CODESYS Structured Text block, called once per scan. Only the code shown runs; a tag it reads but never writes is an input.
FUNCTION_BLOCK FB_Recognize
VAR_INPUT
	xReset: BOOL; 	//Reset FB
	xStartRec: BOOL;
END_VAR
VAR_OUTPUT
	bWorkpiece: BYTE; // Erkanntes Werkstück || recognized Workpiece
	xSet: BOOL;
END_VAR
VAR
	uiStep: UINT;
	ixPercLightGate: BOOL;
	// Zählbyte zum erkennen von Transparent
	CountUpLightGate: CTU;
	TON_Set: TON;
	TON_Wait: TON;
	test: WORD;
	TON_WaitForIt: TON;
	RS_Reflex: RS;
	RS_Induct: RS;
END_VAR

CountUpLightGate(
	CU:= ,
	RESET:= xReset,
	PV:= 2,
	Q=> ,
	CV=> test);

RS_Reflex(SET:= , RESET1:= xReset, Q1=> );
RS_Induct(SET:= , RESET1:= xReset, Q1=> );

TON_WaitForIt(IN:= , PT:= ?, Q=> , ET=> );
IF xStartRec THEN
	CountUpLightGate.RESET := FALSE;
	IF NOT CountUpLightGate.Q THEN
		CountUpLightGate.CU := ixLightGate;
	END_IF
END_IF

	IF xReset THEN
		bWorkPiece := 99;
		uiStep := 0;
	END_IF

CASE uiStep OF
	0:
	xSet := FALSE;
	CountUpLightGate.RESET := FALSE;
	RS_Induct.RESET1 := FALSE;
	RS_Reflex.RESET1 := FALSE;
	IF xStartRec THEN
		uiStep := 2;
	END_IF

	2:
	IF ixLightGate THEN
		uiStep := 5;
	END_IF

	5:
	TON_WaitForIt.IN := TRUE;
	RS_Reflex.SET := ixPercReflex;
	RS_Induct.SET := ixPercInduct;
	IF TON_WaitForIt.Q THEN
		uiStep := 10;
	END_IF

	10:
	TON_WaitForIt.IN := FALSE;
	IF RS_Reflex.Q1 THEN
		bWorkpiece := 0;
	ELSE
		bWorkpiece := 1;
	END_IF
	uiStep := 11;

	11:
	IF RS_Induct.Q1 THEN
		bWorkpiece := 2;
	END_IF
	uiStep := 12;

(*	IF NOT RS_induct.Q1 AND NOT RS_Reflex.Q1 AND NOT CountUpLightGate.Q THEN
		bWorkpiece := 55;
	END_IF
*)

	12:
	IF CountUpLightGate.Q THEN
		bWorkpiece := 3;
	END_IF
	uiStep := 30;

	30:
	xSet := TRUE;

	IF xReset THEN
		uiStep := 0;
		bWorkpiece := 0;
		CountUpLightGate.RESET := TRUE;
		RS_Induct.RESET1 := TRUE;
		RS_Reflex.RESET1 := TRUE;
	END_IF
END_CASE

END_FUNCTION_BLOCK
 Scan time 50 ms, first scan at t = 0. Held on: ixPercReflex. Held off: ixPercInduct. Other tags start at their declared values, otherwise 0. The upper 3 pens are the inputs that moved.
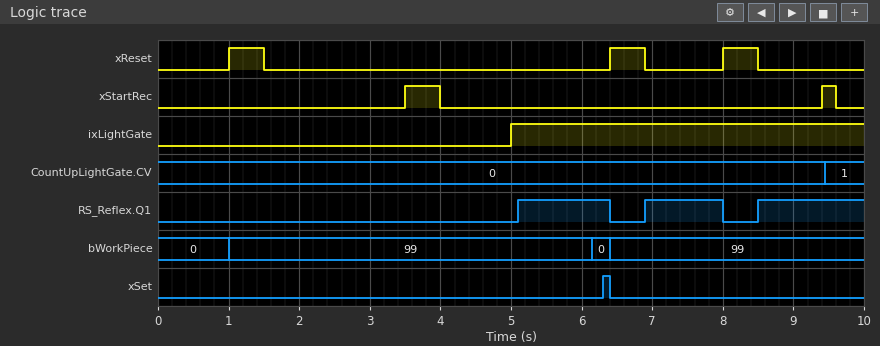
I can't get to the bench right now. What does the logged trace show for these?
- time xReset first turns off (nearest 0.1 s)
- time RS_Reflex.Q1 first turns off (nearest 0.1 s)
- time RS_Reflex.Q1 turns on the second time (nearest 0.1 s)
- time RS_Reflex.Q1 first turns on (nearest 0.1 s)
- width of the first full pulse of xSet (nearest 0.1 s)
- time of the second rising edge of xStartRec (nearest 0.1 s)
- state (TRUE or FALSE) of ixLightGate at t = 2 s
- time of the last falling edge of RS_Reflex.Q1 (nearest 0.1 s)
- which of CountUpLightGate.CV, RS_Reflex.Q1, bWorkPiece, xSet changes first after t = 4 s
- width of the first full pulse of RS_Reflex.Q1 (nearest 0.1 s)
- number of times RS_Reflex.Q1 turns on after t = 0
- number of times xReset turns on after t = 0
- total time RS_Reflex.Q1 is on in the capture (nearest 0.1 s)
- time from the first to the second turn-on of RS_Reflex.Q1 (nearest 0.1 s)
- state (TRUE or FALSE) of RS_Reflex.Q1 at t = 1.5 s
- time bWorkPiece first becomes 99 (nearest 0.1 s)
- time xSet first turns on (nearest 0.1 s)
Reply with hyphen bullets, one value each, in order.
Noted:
- 1.5 s
- 6.4 s
- 6.9 s
- 5.1 s
- 0.1 s
- 9.4 s
- FALSE
- 8.0 s
- RS_Reflex.Q1
- 1.3 s
- 3
- 3
- 3.9 s
- 1.8 s
- FALSE
- 1.0 s
- 6.3 s
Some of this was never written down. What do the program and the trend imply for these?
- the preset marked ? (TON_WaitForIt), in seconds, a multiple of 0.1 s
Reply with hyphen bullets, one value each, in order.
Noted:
- 1.0 s
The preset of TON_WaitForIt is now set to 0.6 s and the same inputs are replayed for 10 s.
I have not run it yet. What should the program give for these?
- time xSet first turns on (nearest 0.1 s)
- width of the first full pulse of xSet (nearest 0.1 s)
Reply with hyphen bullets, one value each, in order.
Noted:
- 5.9 s
- 0.5 s
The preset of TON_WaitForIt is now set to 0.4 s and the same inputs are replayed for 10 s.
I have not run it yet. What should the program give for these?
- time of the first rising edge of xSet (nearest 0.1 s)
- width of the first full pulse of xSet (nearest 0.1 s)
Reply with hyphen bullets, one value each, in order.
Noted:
- 5.7 s
- 0.7 s
